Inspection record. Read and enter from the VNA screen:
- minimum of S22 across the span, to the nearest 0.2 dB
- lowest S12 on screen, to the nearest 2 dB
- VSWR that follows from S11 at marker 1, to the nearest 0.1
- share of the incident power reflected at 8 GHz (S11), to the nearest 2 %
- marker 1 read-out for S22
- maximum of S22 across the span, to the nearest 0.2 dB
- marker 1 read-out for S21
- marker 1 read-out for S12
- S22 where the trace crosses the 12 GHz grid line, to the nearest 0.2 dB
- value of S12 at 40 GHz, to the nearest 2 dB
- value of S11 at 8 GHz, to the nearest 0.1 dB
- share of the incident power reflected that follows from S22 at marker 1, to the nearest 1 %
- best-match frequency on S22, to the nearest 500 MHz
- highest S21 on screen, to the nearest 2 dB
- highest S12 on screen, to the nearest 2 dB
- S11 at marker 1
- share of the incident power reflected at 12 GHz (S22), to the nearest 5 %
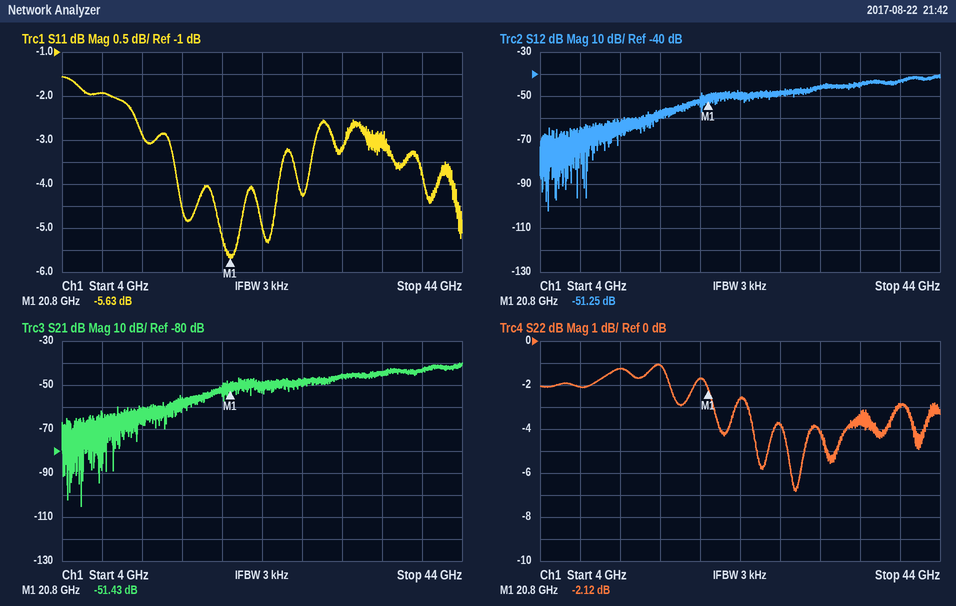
-6.8 dB
-102 dB
3.2
64 %
-2.12 dB
-1.0 dB
-51.43 dB
-51.25 dB
-1.2 dB
-44 dB
-1.9 dB
61 %
29.5 GHz
-40 dB
-40 dB
-5.63 dB
75 %
